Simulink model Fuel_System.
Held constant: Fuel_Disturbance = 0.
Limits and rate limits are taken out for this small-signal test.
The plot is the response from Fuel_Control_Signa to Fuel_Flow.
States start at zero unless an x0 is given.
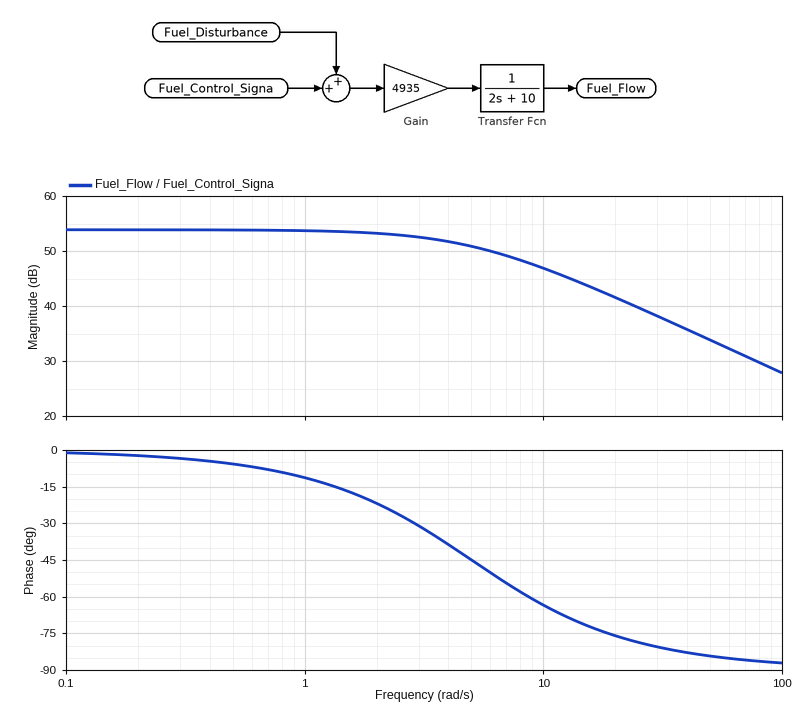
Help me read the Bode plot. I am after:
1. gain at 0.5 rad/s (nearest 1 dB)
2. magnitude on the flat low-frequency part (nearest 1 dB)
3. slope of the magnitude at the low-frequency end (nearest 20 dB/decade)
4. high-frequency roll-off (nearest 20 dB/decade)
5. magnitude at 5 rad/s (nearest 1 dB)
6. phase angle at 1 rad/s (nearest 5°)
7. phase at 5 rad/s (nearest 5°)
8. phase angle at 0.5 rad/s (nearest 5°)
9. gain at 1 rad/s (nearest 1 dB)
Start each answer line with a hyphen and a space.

- 54 dB
- 54 dB
- 0 dB/decade
- -20 dB/decade
- 51 dB
- -10°
- -45°
- -5°
- 54 dB
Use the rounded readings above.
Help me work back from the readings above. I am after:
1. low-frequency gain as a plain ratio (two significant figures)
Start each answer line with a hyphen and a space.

- 500
